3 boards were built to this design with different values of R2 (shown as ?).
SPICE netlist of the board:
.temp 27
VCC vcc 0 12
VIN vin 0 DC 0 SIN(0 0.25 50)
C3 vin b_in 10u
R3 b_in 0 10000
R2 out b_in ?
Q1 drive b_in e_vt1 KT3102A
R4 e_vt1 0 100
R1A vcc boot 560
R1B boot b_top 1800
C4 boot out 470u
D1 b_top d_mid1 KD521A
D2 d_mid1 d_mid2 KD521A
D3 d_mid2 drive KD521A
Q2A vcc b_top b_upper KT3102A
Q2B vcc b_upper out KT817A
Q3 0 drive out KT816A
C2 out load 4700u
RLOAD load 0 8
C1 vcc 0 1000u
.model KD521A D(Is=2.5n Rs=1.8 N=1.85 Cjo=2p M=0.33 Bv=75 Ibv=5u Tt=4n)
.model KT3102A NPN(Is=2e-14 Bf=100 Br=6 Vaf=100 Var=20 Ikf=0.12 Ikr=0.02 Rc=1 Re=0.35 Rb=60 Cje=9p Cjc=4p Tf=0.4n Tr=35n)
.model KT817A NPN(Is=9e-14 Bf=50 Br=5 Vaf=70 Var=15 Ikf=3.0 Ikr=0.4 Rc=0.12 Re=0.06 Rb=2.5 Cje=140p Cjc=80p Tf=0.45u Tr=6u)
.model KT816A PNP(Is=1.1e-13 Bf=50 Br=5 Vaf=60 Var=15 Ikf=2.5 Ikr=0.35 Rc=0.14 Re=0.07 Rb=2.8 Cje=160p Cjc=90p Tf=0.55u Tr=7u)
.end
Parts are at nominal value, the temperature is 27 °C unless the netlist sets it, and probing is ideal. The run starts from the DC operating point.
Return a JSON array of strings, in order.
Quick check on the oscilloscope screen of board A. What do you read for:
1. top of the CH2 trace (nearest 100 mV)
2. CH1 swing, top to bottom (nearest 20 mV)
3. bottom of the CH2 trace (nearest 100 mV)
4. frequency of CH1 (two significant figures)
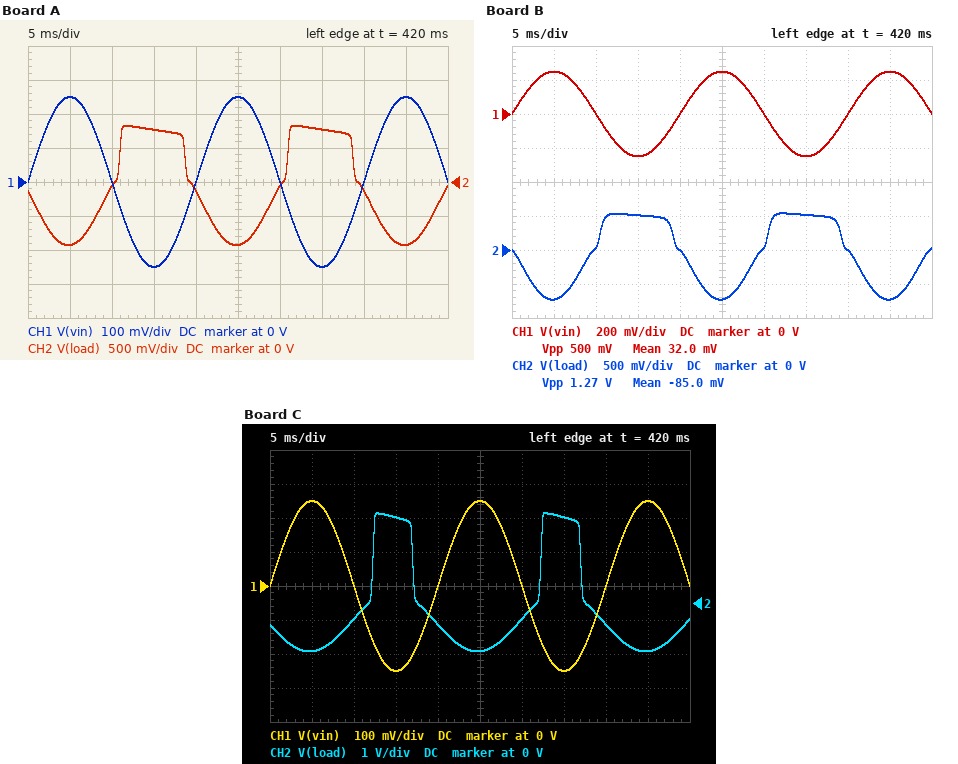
["800 mV", "500 mV", "-900 mV", "50 Hz"]
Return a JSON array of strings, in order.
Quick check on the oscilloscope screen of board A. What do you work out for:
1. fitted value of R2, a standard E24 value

["130 kΩ"]
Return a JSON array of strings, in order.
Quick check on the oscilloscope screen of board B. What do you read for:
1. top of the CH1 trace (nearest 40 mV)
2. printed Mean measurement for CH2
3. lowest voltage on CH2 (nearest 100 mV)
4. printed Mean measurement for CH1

["240 mV", "-85.0 mV", "-700 mV", "32.0 mV"]
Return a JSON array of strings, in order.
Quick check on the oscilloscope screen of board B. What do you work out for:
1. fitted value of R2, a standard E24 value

["150 kΩ"]
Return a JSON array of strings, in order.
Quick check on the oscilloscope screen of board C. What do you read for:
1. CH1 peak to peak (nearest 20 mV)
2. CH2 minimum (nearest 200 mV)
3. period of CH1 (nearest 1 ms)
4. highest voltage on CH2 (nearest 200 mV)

["500 mV", "-1.4 V", "20 ms", "2.6 V"]
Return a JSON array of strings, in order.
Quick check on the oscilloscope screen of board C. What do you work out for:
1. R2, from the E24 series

["68 kΩ"]
